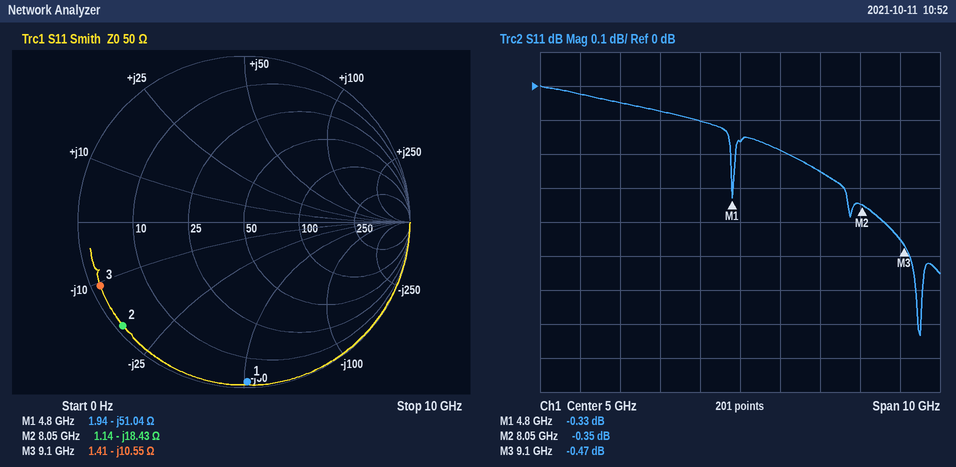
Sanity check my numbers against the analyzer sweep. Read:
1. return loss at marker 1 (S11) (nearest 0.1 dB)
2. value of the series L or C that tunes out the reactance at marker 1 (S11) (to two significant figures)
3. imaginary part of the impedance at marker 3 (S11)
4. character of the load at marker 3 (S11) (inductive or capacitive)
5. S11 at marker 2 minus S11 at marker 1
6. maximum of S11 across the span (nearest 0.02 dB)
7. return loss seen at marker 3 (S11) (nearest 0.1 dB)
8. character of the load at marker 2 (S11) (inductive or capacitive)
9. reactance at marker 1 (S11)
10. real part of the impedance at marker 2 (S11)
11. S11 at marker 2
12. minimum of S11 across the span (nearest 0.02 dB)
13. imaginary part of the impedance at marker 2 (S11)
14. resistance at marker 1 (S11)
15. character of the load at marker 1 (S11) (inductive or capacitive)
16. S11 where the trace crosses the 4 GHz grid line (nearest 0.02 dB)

0.3 dB
1.7 nH
-10.55 Ω
capacitive
-0.02 dB
0.00 dB
0.5 dB
capacitive
-51.04 Ω
1.14 Ω
-0.35 dB
-0.74 dB
-18.43 Ω
1.94 Ω
capacitive
-0.10 dB
